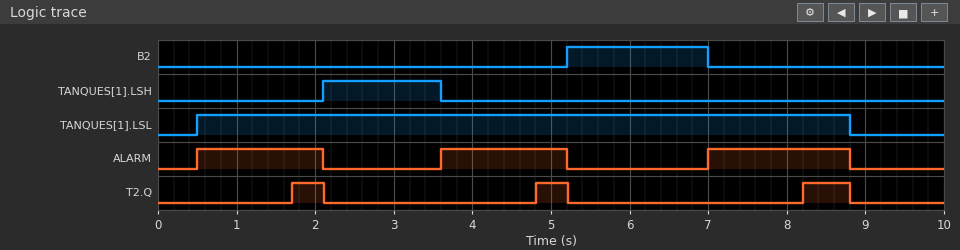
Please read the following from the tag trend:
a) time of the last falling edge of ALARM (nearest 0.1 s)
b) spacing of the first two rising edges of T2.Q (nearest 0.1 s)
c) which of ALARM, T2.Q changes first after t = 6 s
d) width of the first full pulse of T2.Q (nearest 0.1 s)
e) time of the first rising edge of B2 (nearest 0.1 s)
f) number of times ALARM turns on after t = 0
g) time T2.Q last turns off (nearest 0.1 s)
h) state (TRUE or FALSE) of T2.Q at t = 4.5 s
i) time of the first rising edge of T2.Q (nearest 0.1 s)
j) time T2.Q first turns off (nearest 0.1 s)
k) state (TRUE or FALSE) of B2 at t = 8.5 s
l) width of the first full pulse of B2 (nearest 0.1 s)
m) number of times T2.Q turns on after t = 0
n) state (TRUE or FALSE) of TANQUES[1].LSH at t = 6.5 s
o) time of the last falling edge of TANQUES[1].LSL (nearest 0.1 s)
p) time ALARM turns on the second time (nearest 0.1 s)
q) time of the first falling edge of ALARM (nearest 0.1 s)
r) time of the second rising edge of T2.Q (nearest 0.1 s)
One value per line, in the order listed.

8.8 s
3.1 s
ALARM
0.4 s
5.2 s
3
8.8 s
FALSE
1.7 s
2.1 s
FALSE
1.8 s
3
FALSE
8.8 s
3.6 s
2.1 s
4.8 s
